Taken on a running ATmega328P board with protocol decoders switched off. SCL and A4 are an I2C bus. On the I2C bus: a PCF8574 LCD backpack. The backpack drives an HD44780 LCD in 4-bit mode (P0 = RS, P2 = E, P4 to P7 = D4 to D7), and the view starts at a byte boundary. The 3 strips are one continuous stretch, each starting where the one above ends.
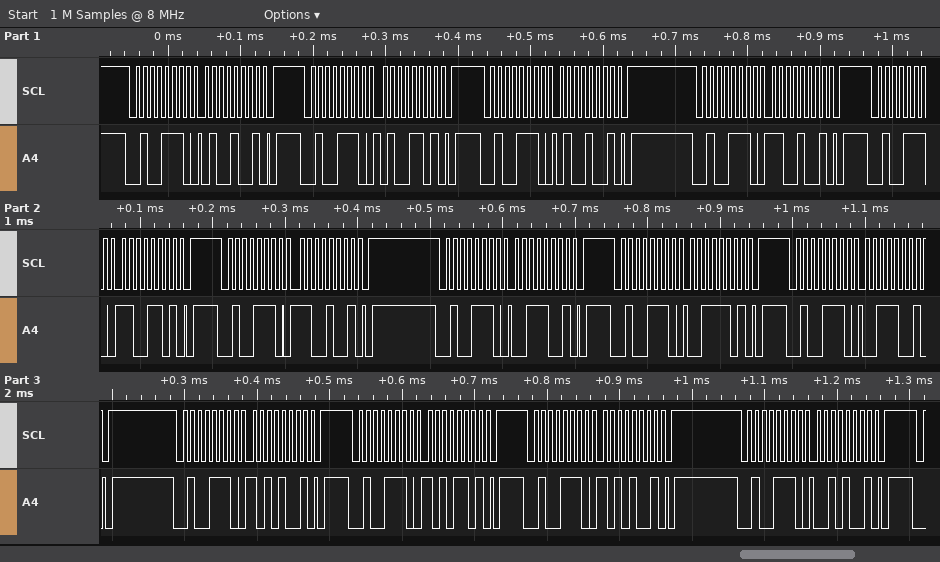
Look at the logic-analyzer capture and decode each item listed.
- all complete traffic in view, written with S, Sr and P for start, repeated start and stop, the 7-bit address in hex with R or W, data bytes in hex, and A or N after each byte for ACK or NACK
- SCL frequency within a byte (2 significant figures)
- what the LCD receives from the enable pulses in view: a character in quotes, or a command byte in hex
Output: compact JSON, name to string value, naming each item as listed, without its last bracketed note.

{"all complete traffic in view, written with S, Sr and P for start, repeated start and stop, the 7-bit address in hex with R or W, data bytes in hex, and A or N after each byte for ACK or NACK": "S 27W A 49 A P S 27W A 4D A P S 27W A 49 A P S 27W A C9 A P S 27W A CD A P S 27W A C9 A P S 27W A 39 A P S 27W A 3D A P S 27W A 39 A P S 27W A A9 A P S 27W A AD A P S 27W A A9 A P S 27W A 29 A P", "SCL frequency within a byte": "100 kHz", "what the LCD receives from the enable pulses in view: a character in quotes, or a command byte in hex": "'L' ':'"}
